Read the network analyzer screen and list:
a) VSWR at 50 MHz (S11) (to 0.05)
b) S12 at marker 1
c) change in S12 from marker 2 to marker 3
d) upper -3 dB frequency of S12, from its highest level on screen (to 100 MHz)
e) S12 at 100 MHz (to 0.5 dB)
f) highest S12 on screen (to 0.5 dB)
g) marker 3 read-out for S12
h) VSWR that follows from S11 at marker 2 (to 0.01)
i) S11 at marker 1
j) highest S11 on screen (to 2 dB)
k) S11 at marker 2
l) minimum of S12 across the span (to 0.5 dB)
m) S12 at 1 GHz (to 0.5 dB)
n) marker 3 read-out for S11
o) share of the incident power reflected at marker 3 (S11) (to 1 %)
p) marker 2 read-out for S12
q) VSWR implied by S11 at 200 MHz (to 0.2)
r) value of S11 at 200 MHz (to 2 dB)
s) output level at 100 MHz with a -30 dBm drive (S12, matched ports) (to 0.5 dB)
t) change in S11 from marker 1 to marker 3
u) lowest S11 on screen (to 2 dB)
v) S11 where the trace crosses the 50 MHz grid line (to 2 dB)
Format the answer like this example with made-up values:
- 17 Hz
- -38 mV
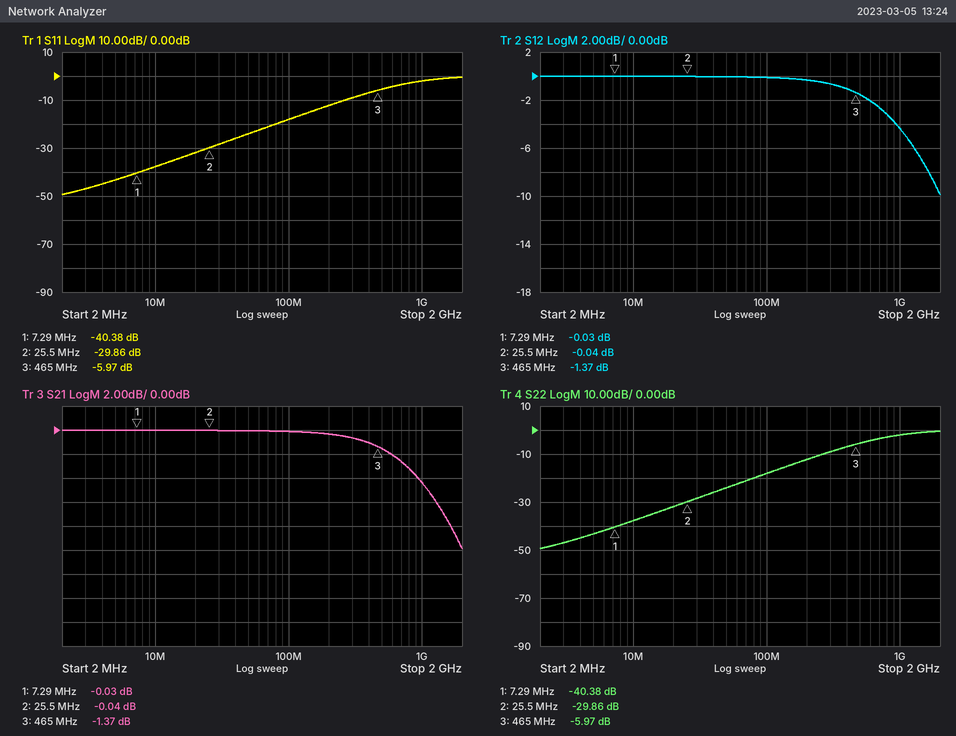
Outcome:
- 1.15
- -0.03 dB
- -1.33 dB
- 800 MHz
- 0.0 dB
- 0.0 dB
- -1.37 dB
- 1.07
- -40.38 dB
- 0 dB
- -29.86 dB
- -10.0 dB
- -4.5 dB
- -5.97 dB
- 25 %
- -0.04 dB
- 1.6
- -12 dB
- -30.0 dBm
- 34.41 dB
- -50 dB
- -24 dB
